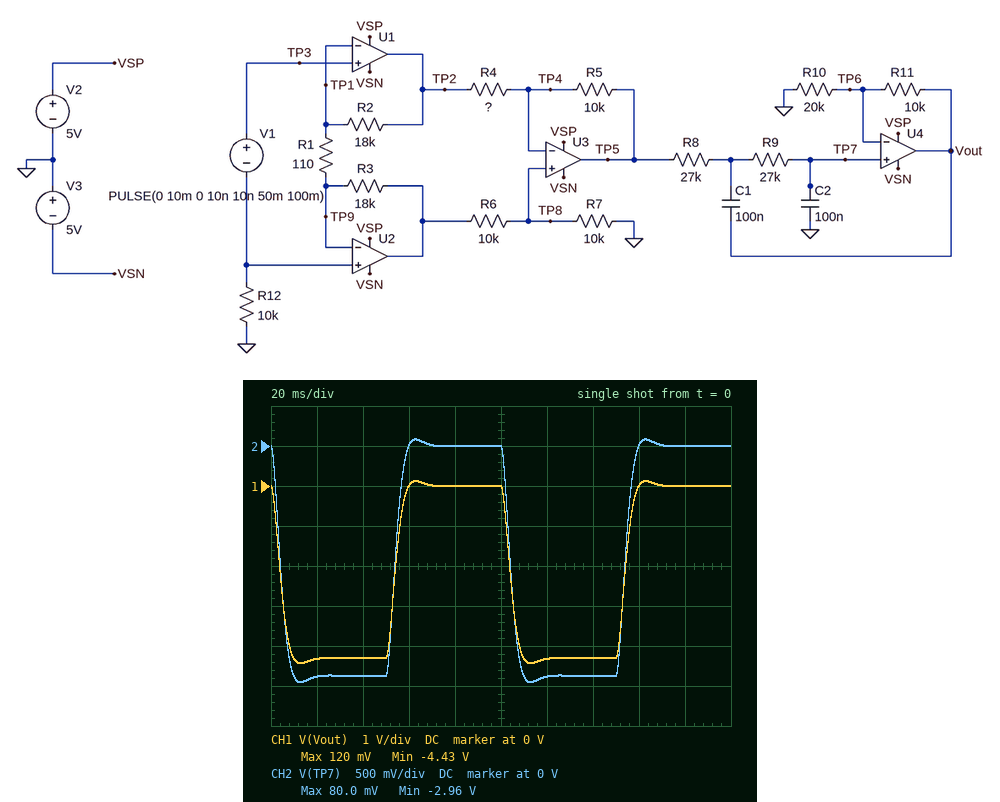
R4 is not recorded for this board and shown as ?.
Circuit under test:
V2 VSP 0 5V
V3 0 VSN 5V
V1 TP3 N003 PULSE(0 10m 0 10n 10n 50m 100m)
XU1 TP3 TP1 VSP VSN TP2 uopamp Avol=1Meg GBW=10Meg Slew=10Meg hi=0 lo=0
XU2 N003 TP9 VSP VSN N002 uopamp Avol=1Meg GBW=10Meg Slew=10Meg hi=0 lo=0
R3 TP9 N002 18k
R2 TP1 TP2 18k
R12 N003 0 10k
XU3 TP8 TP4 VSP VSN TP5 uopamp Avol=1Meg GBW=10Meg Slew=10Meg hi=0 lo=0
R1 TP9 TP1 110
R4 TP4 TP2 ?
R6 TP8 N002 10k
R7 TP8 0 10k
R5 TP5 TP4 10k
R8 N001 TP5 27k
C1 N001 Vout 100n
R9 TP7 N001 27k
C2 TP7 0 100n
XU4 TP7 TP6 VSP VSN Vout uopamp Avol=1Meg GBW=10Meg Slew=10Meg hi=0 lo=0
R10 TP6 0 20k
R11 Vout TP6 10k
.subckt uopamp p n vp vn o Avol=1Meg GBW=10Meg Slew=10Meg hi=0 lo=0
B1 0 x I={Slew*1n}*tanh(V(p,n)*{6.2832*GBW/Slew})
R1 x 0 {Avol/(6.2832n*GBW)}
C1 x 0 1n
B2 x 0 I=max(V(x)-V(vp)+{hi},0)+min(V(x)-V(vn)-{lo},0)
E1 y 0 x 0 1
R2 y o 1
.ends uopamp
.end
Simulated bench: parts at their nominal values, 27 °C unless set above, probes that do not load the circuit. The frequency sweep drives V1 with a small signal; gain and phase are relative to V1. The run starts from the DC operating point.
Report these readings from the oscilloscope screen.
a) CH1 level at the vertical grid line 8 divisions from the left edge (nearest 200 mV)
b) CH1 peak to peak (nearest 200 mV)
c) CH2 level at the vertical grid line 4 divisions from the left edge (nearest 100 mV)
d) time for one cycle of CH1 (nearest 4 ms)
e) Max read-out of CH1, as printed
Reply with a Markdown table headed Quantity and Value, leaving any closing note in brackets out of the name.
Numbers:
| Quantity | Value |
|---|---|
| CH1 level at the vertical grid line 8 divisions from the left edge | 0 V |
| CH1 peak to peak | 4.6 V |
| CH2 level at the vertical grid line 4 divisions from the left edge | 0 V |
| time for one cycle of CH1 | 100 ms |
| Max read-out of CH1, as printed | 120 mV |
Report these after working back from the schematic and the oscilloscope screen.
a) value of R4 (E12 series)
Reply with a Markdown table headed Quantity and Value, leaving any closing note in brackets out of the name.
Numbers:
| Quantity | Value |
|---|---|
| value of R4 | 12 kΩ |
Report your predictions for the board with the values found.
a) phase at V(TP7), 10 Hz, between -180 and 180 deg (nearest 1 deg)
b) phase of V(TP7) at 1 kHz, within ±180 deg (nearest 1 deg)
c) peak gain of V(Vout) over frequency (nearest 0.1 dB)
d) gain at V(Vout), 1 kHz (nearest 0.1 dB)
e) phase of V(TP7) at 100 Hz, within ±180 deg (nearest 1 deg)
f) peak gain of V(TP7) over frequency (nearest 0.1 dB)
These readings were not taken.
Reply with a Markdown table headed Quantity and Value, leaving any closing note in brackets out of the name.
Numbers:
| Quantity | Value |
|---|---|
| phase at V(TP7), 10 Hz, between -180 and 180 deg | 165 deg |
| phase of V(TP7) at 1 kHz, within ±180 deg | 3 deg |
| peak gain of V(Vout) over frequency | 52.7 dB |
| gain at V(Vout), 1 kHz | 3.5 dB |
| phase of V(TP7) at 100 Hz, within ±180 deg | 53 deg |
| peak gain of V(TP7) over frequency | 49.2 dB |
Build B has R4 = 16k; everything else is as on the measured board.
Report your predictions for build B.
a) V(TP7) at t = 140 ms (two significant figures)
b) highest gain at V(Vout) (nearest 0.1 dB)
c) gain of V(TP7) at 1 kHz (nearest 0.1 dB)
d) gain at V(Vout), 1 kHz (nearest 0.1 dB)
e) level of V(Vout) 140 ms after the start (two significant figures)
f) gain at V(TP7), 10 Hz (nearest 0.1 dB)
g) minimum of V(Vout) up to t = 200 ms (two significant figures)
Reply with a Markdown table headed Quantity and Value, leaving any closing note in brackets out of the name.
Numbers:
| Quantity | Value |
|---|---|
| V(TP7) at t = 140 ms | -2.4 V |
| highest gain at V(Vout) | 51.0 dB |
| gain of V(TP7) at 1 kHz | -1.7 dB |
| gain at V(Vout), 1 kHz | 1.8 dB |
| level of V(Vout) 140 ms after the start | -3.5 V |
| gain at V(TP7), 10 Hz | 47.4 dB |
| minimum of V(Vout) up to t = 200 ms | -3.6 V |
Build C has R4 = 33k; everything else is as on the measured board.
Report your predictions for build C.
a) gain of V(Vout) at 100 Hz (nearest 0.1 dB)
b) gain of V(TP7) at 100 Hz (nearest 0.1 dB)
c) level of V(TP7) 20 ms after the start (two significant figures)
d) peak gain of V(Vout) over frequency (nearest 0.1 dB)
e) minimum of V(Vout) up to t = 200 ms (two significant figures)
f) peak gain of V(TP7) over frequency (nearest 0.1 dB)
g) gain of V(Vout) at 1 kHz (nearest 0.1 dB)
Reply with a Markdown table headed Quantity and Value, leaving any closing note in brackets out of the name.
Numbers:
| Quantity | Value |
|---|---|
| gain of V(Vout) at 100 Hz | 37.4 dB |
| gain of V(TP7) at 100 Hz | 33.9 dB |
| level of V(TP7) 20 ms after the start | -1.6 V |
| peak gain of V(Vout) over frequency | 47.4 dB |
| minimum of V(Vout) up to t = 200 ms | -2.4 V |
| peak gain of V(TP7) over frequency | 43.9 dB |
| gain of V(Vout) at 1 kHz | -1.8 dB |
